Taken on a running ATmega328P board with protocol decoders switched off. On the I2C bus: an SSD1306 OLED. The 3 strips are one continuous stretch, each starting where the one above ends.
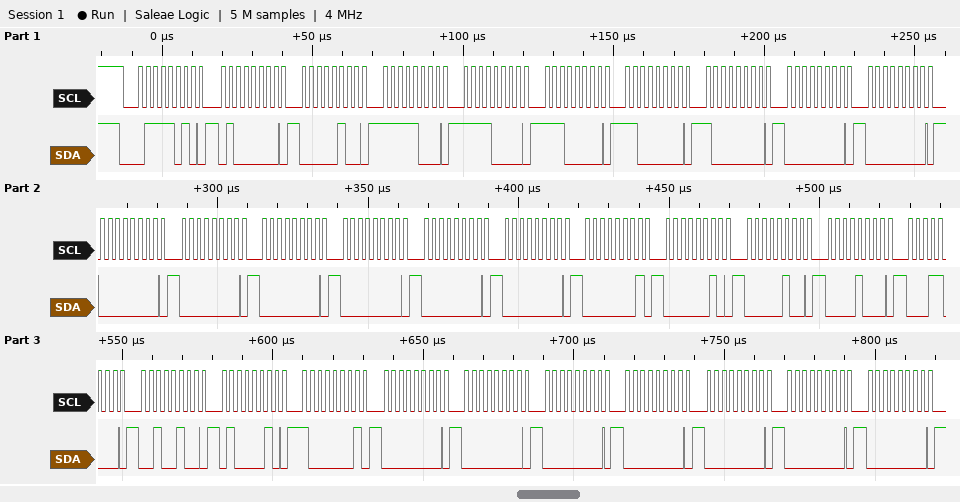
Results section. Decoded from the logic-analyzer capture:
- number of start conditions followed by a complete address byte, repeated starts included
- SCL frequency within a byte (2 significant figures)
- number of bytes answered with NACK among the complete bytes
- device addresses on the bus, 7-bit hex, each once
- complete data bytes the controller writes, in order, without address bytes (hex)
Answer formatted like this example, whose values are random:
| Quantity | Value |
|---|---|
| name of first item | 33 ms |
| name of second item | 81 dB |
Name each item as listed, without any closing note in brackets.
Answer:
| Quantity | Value |
|---|---|
| number of start conditions followed by a complete address byte, repeated starts included | 1 |
| SCL frequency within a byte | 400 kHz |
| number of bytes answered with NACK among the complete bytes | 0 |
| device addresses on the bus, 7-bit hex, each once | 0x3D |
| complete data bytes the controller writes, in order, without address bytes | 40 04 F8 F0 E0 C0 80 00 00 00 00 00 00 00 00 01 02 04 08 18 24 42 81 00 00 00 00 00 00 00 |
